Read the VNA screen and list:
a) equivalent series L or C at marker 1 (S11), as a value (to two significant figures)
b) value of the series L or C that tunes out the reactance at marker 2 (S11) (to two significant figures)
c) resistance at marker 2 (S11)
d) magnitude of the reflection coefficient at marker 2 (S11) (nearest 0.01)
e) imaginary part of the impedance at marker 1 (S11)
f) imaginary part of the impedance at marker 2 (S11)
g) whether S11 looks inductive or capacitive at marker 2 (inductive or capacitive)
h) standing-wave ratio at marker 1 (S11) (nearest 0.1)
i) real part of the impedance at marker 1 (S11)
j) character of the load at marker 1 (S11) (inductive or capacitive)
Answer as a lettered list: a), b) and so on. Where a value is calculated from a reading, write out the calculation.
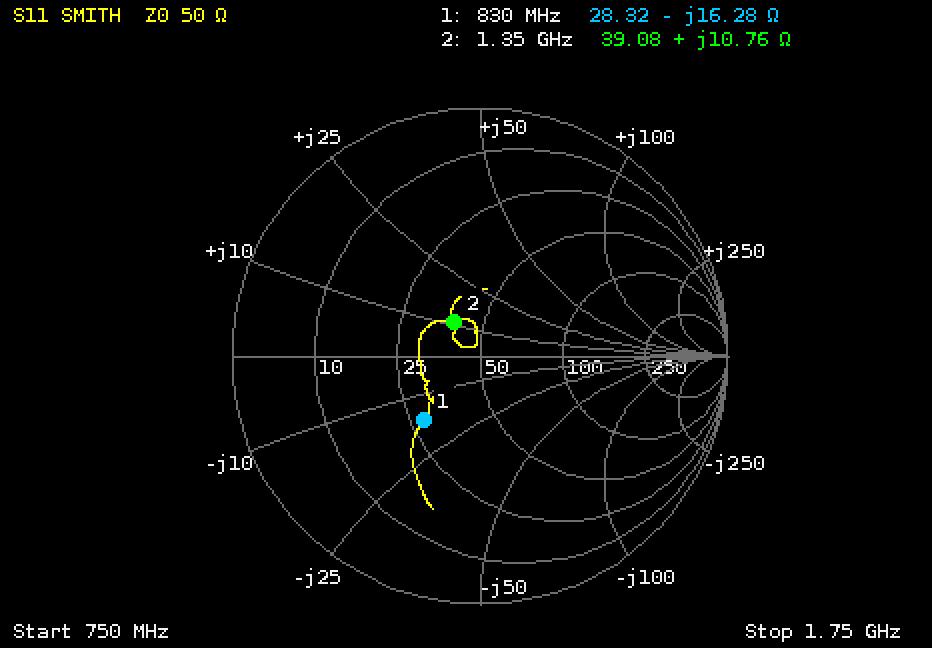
a) C = 1/(2π × 830 MHz × 16.28 Ω) ≈ 12 pF
b) C = 1/(2π × 1.35 GHz × 10.76 Ω) ≈ 11 pF
c) 39.08 Ω
d) 0.17
e) -16.28 Ω
f) +10.76 Ω
g) inductive
h) 2.0
i) 28.32 Ω
j) capacitive
